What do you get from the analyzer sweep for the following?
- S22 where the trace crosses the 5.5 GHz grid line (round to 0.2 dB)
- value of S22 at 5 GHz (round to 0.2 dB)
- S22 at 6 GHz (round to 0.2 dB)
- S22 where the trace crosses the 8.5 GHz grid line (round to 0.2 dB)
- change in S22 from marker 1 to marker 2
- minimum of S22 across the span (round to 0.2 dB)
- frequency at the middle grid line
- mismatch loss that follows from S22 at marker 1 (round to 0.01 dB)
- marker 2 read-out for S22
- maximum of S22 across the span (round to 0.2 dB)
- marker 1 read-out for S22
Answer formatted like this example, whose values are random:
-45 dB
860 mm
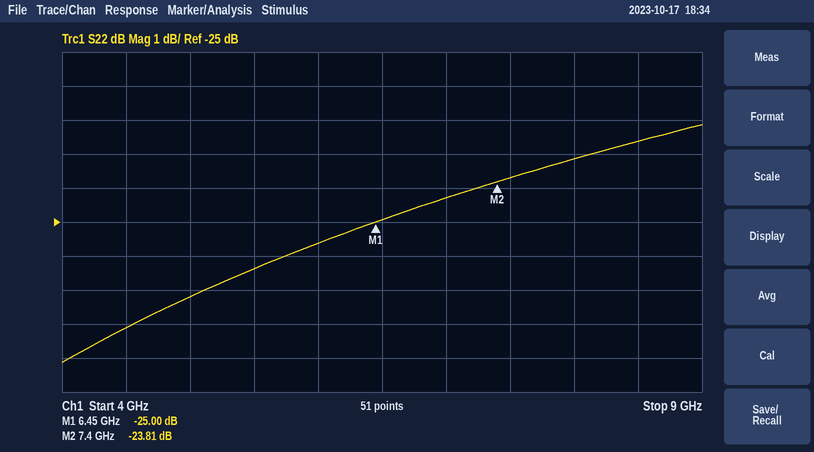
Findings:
-26.4 dB
-27.2 dB
-25.6 dB
-22.6 dB
1.19 dB
-29.2 dB
6.5 GHz
0.01 dB
-23.81 dB
-22.2 dB
-25.00 dB
